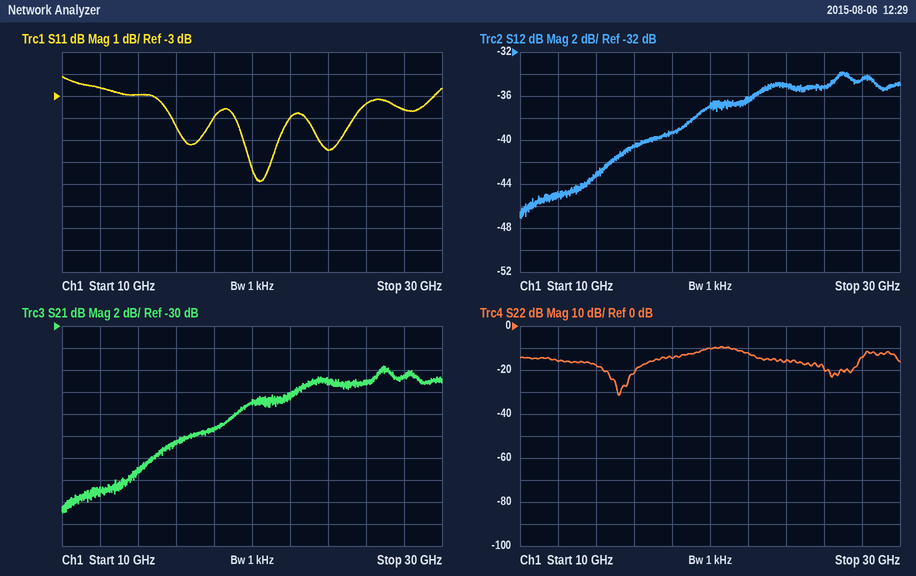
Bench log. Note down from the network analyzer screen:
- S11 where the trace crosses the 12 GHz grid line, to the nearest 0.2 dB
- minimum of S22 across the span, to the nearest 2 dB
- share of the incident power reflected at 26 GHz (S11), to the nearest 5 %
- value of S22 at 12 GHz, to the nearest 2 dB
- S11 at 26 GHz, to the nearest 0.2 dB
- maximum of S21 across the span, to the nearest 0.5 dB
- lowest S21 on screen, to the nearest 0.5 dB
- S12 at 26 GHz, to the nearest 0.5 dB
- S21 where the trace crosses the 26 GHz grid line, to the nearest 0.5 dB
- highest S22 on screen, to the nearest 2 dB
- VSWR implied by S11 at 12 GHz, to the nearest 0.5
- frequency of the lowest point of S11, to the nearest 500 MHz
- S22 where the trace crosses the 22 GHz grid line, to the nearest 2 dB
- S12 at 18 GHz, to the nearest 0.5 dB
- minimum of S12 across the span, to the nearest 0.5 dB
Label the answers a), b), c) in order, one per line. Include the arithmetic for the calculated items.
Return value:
a) -2.6 dB
b) -32 dB
c) 10^(-3.4/10) ≈ 45.7 %, so 45 % to the nearest 5 %
d) -16 dB
e) -3.4 dB
f) -33.5 dB
g) -47.0 dB
h) -35.0 dB
i) -35.0 dB
j) -10 dB
k) |Γ| = 10^(-2.6/20) = 0.7413; VSWR = (1 + 0.7413)/(1 − 0.7413) ≈ 6.73, so 6.5 to the nearest 0.5
l) 20.5 GHz
m) -12 dB
n) -39.5 dB
o) -47.0 dB
